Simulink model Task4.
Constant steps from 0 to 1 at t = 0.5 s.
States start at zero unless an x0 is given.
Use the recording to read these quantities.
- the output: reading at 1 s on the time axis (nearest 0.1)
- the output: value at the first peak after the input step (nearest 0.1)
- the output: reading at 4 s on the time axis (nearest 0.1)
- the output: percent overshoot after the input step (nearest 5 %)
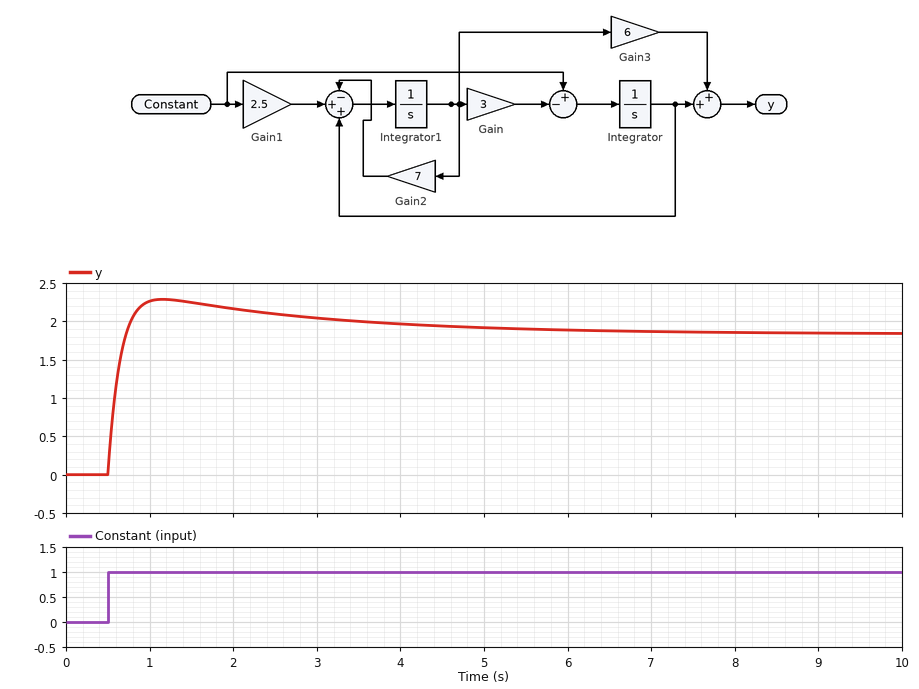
2.3
2.3
2.0
25 %
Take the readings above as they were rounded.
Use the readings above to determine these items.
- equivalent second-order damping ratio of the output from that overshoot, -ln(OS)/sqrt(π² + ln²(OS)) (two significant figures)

0.40
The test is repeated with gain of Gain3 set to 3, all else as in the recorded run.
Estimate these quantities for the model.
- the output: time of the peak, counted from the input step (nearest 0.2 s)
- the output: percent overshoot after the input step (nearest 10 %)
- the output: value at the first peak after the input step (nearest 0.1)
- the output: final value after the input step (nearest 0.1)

0.6 s
40 %
1.2
0.8
